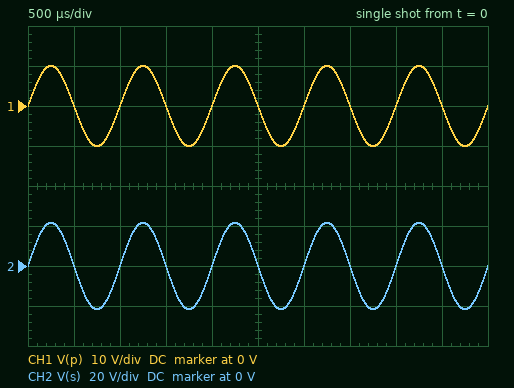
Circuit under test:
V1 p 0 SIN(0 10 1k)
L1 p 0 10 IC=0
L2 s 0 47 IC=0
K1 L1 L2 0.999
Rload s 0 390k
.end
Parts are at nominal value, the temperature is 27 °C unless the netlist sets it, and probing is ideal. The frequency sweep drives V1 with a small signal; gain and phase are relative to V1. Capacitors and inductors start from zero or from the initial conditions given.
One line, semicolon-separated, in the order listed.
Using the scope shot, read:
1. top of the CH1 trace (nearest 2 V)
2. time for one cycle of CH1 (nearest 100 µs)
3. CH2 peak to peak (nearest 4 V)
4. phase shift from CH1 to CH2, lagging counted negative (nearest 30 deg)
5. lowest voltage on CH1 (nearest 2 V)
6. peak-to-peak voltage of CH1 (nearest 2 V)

10 V; 1.0 ms; 44 V; 0 deg; -10 V; 20 V
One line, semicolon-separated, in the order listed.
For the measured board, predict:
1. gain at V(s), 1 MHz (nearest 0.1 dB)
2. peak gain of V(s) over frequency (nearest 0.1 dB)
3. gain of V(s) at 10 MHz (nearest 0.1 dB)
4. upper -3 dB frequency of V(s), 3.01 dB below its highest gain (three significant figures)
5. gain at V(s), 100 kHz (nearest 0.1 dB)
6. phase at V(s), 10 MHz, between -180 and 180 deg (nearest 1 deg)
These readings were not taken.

1.5 dB; 6.7 dB; -16.9 dB; 661 kHz; 6.6 dB; -86 deg
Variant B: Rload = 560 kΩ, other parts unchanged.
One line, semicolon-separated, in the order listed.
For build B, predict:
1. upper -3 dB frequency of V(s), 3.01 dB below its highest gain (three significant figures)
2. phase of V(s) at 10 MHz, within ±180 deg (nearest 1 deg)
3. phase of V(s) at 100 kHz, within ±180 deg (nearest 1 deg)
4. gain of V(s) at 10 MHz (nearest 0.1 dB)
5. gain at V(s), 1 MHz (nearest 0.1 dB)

949 kHz; -85 deg; -6 deg; -13.8 dB; 3.5 dB
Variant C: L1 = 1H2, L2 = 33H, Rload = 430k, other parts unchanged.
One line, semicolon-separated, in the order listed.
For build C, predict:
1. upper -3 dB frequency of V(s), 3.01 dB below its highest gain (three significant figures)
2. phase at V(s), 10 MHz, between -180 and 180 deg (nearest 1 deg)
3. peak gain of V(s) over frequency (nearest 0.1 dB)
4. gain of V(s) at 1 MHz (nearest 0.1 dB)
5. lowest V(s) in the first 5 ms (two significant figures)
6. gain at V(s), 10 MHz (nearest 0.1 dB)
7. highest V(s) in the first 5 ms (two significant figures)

1.04 MHz; -84 deg; 14.4 dB; 11.5 dB; -52 V; -5.3 dB; 52 V
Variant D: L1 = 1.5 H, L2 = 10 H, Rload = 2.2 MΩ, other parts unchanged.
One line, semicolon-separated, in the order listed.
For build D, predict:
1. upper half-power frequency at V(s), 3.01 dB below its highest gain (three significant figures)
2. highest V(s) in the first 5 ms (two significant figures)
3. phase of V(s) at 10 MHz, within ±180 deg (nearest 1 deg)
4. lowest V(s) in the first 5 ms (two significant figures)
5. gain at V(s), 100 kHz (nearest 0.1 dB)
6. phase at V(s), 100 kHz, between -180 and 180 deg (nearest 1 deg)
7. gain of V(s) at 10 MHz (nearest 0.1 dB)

17.5 MHz; 26 V; -30 deg; -26 V; 8.2 dB; 0 deg; 7.0 dB
